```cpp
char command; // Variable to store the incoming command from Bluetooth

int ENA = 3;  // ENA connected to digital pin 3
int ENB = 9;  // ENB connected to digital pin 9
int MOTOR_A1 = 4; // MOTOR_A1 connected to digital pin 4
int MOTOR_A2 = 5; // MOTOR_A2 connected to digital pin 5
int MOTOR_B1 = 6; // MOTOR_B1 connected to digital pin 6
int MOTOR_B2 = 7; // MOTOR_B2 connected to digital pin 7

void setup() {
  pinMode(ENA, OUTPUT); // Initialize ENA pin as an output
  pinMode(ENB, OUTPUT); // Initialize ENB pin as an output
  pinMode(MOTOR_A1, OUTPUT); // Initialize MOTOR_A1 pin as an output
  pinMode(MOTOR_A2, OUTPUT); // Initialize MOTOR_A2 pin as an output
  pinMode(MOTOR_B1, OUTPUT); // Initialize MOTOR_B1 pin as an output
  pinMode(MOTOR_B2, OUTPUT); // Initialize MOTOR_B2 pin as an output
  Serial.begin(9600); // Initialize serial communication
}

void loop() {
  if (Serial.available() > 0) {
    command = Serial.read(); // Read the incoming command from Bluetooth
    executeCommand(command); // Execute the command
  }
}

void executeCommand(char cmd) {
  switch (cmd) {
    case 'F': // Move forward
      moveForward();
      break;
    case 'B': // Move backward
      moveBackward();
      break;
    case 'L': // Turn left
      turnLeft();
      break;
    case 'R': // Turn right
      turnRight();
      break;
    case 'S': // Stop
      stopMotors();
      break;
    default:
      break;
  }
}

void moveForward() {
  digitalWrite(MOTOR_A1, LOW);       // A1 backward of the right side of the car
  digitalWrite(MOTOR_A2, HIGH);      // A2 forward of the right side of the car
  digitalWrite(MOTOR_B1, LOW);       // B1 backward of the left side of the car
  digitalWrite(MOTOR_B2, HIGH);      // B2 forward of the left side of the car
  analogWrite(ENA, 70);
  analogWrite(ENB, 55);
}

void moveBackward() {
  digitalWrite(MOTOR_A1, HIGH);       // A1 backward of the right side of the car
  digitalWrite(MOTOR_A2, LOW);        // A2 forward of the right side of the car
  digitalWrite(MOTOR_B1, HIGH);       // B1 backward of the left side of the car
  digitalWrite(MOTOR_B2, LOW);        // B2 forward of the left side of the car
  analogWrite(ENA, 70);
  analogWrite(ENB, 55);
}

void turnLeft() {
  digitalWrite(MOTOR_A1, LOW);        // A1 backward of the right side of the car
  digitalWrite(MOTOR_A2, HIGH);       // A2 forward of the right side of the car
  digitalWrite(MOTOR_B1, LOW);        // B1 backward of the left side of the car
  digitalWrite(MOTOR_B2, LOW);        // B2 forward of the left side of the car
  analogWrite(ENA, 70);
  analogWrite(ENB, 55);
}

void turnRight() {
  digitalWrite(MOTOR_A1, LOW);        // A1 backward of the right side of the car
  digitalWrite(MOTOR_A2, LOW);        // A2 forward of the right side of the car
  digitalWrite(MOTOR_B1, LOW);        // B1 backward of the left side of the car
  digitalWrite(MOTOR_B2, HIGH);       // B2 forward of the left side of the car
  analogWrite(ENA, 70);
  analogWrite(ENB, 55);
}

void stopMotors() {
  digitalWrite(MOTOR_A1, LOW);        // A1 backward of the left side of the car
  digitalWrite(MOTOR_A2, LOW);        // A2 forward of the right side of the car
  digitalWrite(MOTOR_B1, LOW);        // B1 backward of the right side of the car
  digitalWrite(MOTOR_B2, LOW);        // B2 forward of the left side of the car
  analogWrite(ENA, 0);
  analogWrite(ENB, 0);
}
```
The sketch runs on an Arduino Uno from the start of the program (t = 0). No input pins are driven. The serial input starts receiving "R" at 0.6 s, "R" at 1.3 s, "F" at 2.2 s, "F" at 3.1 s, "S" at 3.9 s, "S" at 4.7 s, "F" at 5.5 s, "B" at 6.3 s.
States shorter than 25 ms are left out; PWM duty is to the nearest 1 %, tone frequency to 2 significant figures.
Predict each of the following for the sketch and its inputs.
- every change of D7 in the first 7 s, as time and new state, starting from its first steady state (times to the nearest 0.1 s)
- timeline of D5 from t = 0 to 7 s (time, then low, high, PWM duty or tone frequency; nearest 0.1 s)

0 s low; 0.6 s high; 3.9 s low; 5.5 s high; 6.3 s low
0 s low; 2.2 s high; 3.9 s low; 5.5 s high; 6.3 s low
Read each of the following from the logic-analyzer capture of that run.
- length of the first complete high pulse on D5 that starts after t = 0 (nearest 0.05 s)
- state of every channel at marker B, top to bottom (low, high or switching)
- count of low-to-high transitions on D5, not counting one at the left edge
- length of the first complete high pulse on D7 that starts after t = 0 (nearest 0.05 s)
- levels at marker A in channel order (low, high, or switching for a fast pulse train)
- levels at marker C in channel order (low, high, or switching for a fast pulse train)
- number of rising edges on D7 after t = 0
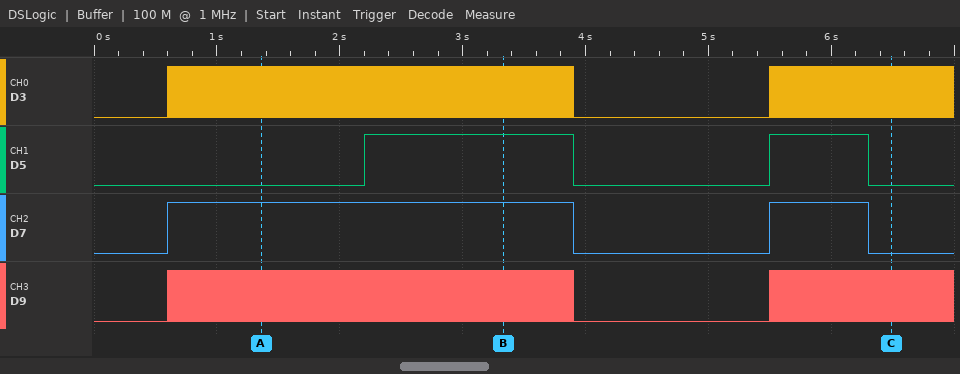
1.70 s
D3 switching, D5 high, D7 high, D9 switching
2
3.30 s
D3 switching, D5 low, D7 high, D9 switching
D3 switching, D5 low, D7 low, D9 switching
2
